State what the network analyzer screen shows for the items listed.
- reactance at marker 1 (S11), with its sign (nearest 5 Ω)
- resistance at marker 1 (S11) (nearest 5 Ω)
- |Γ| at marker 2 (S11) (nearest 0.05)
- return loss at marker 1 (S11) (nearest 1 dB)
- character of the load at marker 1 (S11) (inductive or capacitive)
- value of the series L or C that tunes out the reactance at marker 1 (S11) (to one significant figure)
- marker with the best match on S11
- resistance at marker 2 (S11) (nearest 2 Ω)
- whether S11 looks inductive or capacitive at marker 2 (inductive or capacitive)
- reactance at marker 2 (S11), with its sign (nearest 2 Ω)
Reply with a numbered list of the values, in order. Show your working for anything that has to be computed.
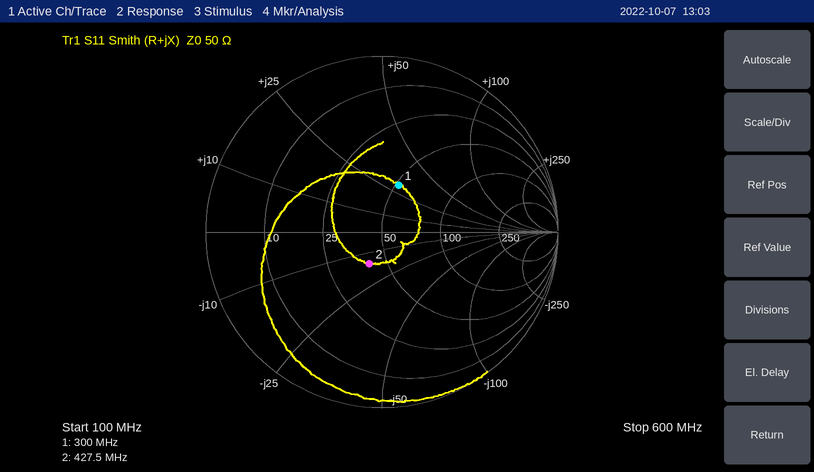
1. +30 Ω
2. 50 Ω
3. 0.20
4. 11 dB
5. inductive
6. C = 1/(2π × 300 MHz × 30 Ω) ≈ 17.7 pF, so 20 pF to one significant figure
7. marker 2
8. 40 Ω
9. capacitive
10. -16 Ω
